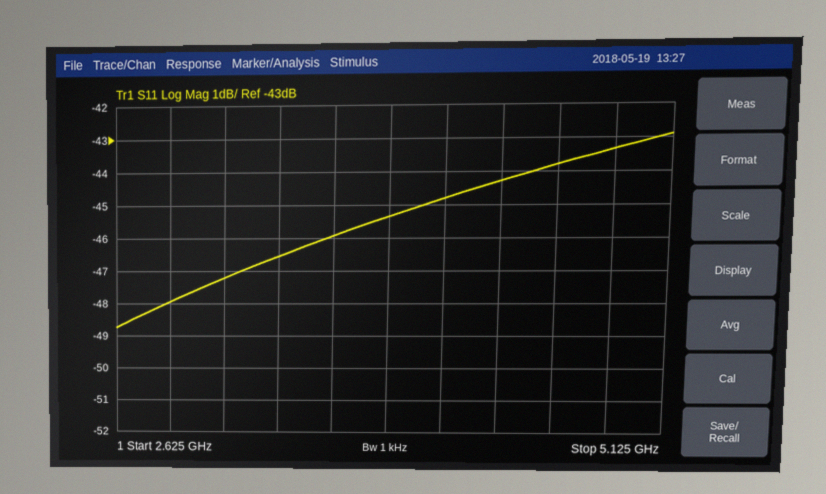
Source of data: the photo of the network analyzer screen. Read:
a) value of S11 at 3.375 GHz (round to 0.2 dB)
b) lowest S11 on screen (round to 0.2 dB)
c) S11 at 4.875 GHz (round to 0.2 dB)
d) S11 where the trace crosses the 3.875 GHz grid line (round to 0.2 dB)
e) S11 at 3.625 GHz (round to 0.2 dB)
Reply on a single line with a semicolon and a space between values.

-46.6 dB; -48.8 dB; -43.4 dB; -45.4 dB; -46.0 dB
